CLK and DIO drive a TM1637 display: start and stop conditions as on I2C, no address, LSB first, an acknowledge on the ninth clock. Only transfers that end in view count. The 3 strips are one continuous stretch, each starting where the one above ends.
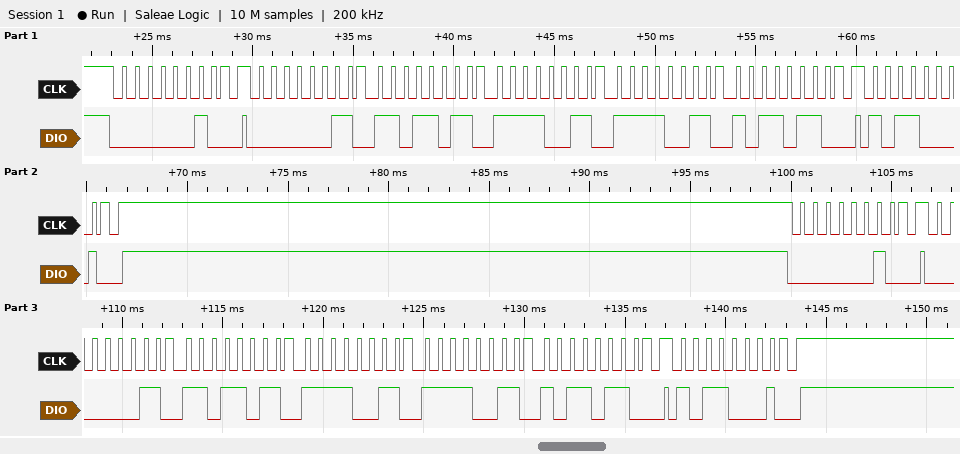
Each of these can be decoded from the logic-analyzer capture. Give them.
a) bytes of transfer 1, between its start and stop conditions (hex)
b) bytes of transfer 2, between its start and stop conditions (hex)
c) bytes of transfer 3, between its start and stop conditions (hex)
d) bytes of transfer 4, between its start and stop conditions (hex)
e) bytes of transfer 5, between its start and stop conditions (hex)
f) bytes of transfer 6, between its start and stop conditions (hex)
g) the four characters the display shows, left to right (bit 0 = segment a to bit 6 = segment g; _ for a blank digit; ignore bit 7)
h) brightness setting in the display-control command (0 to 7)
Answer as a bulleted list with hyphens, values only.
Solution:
- 40
- C0 DB CF CF 6D
- 8D
- 40
- C0 DB CF CF 6D
- 8D
- 2335
- 5
